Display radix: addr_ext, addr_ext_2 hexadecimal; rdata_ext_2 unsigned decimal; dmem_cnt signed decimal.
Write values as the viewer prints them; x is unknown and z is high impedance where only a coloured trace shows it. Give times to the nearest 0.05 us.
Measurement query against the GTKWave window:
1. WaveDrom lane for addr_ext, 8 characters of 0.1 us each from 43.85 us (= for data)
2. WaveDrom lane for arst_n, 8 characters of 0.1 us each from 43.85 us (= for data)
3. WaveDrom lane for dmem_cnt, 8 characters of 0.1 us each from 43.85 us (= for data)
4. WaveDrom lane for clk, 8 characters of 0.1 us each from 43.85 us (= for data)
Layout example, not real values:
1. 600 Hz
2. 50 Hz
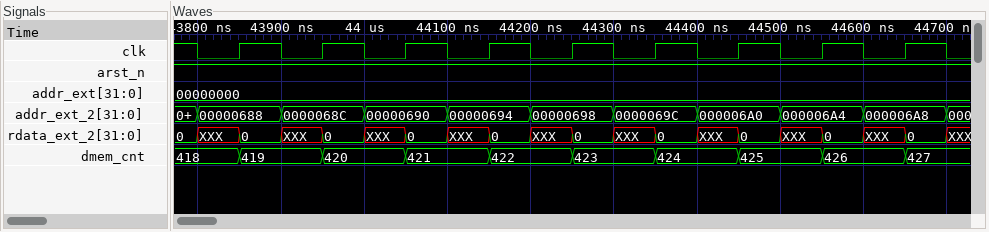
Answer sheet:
1. {name: 'addr_ext', wave: '=.......', data: '00000000'}
2. {name: 'arst_n', wave: '1.......'}
3. {name: 'dmem_cnt', wave: '========', data: '419 420 421 422 423 424 425 426'}
4. {name: 'clk', wave: 'p.......'}
